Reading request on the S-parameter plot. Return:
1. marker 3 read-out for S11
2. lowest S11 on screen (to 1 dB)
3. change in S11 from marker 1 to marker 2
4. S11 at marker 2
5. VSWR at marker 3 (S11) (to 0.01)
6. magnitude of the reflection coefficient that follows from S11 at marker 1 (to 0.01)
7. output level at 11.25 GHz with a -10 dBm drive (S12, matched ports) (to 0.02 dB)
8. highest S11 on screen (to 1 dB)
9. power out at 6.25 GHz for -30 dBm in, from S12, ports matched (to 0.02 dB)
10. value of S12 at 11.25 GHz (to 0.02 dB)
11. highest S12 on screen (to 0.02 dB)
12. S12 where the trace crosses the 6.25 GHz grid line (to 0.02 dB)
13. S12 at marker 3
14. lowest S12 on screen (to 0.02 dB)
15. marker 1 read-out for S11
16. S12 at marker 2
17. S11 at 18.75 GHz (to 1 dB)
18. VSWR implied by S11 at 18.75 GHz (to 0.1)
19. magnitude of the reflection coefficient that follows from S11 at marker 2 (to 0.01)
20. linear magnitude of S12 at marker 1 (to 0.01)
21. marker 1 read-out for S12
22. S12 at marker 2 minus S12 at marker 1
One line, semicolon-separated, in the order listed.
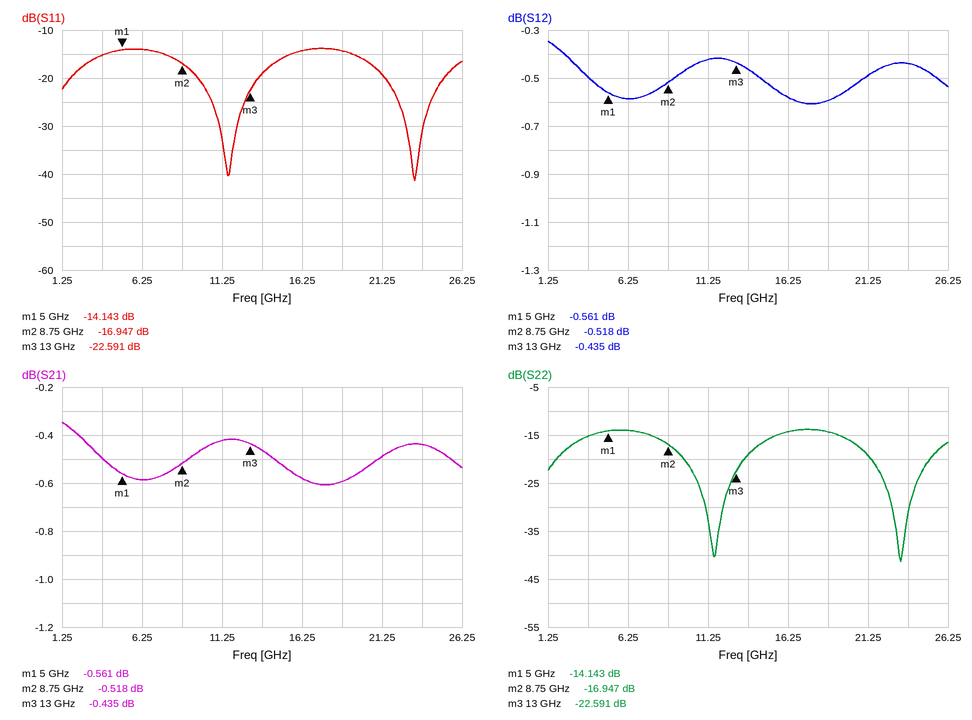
-22.591 dB; -41 dB; -2.804 dB; -16.947 dB; 1.16; 0.20; -10.42 dBm; -14 dB; -30.58 dBm; -0.42 dB; -0.34 dB; -0.58 dB; -0.435 dB; -0.60 dB; -14.143 dB; -0.518 dB; -14 dB; 1.5; 0.14; 0.94; -0.561 dB; 0.043 dB
